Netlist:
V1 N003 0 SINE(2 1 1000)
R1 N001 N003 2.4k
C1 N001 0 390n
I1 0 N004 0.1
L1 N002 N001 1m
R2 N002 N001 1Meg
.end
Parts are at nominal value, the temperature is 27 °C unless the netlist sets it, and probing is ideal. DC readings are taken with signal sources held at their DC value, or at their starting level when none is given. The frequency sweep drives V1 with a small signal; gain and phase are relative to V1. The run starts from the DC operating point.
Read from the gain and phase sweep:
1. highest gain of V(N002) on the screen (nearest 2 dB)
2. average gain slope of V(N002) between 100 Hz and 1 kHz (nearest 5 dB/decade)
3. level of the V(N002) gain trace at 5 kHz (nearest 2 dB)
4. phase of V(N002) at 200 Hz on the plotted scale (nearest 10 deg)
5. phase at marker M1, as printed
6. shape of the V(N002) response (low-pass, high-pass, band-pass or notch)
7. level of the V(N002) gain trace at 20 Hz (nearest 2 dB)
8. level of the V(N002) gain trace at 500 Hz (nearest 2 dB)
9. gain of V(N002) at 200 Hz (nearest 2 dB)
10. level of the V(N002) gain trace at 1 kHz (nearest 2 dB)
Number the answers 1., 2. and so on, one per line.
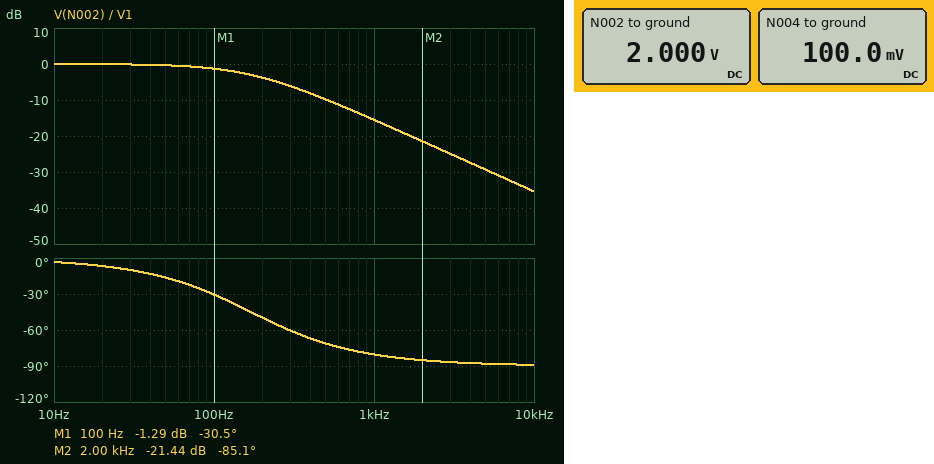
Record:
1. 0 dB
2. -15 dB/decade
3. -30 dB
4. -50 deg
5. -30.5 deg
6. low-pass
7. 0 dB
8. -10 dB
9. -4 dB
10. -16 dB
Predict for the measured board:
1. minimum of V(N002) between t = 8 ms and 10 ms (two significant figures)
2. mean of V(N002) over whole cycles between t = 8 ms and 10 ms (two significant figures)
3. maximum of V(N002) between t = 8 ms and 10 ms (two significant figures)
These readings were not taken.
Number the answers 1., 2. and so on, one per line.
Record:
1. 1.8 V
2. 2.0 V
3. 2.2 V
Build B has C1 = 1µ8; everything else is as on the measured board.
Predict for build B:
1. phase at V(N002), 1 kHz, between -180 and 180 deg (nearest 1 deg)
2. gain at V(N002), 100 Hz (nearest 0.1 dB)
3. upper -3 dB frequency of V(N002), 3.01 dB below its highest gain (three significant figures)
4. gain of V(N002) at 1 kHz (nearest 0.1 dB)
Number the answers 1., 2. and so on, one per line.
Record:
1. -88 deg
2. -9.2 dB
3. 36.8 Hz
4. -28.7 dB
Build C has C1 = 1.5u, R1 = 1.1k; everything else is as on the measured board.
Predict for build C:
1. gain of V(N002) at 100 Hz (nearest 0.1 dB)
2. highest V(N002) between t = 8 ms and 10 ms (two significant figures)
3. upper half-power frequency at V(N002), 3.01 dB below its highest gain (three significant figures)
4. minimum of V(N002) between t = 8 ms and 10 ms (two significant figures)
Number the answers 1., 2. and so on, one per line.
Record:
1. -3.2 dB
2. 2.1 V
3. 96.5 Hz
4. 1.9 V
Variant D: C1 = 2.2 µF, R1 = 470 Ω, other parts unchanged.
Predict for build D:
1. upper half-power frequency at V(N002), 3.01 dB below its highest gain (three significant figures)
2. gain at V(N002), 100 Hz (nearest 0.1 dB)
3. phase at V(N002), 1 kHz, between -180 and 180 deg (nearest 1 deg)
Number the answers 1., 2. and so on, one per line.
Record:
1. 154 Hz
2. -1.5 dB
3. -81 deg
